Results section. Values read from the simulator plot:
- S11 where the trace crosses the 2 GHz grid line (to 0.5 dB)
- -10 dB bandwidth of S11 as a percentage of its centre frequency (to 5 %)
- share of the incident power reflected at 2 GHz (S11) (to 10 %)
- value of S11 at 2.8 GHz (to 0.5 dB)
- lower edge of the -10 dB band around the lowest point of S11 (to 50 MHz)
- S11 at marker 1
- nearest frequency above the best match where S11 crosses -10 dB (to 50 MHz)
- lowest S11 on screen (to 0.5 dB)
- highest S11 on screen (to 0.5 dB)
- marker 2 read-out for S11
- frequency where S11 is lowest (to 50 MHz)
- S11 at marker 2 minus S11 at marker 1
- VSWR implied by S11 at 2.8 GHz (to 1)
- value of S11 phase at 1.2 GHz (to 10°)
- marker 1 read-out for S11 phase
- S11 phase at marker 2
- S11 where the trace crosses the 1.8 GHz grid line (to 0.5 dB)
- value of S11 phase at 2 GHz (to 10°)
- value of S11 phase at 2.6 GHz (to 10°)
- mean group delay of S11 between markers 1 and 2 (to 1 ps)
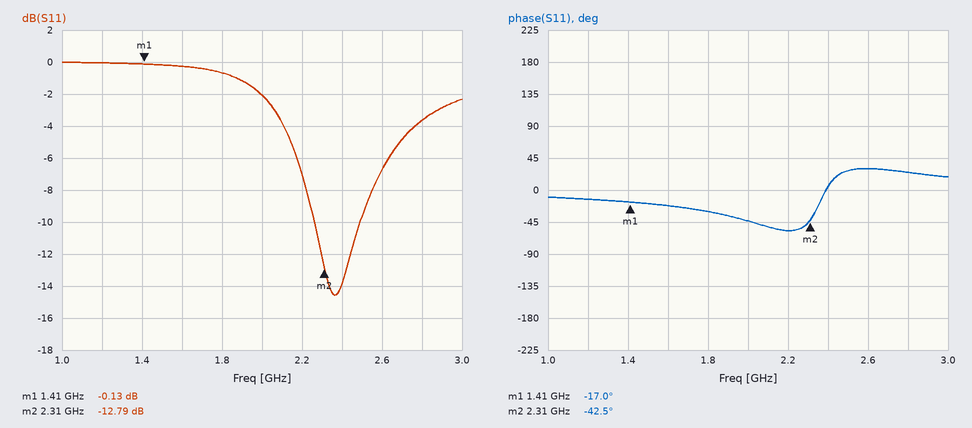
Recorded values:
-2.0 dB
10 %
60 %
-3.5 dB
2.25 GHz
-0.13 dB
2.50 GHz
-14.5 dB
0.0 dB
-12.79 dB
2.35 GHz
-12.66 dB
5
-10°
-17.0°
-42.5°
-0.5 dB
-40°
30°
79 ps
